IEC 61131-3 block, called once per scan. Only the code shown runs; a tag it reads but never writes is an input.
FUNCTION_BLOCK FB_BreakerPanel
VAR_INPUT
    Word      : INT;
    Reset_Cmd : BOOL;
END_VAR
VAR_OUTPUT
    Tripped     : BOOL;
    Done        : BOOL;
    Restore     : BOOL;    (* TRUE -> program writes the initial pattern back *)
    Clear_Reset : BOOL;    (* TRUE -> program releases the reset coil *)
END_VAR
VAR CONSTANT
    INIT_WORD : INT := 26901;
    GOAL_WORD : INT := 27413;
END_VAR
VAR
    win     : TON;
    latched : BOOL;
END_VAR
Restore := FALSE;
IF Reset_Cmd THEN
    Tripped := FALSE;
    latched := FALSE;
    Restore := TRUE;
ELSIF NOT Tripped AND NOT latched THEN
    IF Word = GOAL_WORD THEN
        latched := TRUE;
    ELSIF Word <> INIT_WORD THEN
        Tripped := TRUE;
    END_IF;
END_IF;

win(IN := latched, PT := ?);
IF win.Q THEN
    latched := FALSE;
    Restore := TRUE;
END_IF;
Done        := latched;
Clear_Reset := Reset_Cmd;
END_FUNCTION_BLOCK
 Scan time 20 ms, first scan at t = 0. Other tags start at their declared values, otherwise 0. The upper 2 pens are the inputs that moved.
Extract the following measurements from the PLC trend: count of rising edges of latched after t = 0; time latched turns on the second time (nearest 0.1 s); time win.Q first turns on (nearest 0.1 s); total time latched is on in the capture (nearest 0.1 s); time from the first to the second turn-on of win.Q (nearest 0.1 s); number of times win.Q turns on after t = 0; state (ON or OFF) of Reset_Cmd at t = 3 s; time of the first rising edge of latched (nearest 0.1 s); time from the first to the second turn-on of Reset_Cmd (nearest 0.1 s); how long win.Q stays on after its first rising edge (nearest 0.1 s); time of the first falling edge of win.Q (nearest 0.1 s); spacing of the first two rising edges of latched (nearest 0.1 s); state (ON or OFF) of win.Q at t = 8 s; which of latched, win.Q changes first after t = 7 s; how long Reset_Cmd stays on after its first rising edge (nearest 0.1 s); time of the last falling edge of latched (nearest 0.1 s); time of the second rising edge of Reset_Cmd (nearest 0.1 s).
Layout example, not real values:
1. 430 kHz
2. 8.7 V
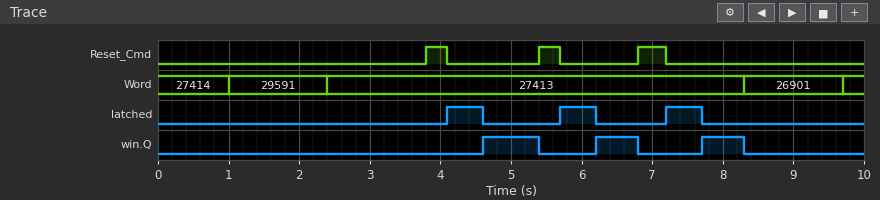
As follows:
1. 3
2. 5.7 s
3. 4.6 s
4. 1.5 s
5. 1.6 s
6. 3
7. OFF
8. 4.1 s
9. 1.6 s
10. 0.8 s
11. 5.4 s
12. 1.6 s
13. ON
14. latched
15. 0.3 s
16. 7.7 s
17. 5.4 s
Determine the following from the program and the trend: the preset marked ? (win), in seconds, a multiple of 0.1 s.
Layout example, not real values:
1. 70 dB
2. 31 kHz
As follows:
1. 0.5 s
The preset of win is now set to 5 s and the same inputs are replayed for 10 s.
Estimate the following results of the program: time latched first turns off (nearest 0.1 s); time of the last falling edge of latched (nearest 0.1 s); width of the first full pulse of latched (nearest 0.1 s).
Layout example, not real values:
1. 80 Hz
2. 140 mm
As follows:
1. 5.4 s
2. 6.8 s
3. 1.3 s
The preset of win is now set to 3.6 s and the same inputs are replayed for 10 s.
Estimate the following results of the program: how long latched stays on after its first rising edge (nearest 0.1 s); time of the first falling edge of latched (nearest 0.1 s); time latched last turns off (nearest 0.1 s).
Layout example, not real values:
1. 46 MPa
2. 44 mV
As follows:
1. 1.3 s
2. 5.4 s
3. 6.8 s
